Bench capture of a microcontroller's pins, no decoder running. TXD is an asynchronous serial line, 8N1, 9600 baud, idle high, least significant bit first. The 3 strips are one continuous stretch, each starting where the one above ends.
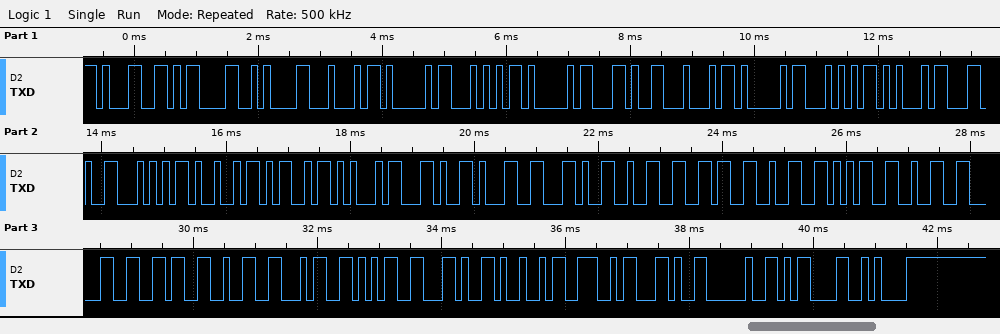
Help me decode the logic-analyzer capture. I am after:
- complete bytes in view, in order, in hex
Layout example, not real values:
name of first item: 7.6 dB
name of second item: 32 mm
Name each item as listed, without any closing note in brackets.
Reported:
complete bytes in view, in order, in hex: 31 0D 0A 44 41 54 41 2C 44 41 54 45 2C 54 49 4D 45 2C 31 2C 32 36 32 35 32 30 36 32 34 35 2C 49 4E 2C 20 0D 0A
